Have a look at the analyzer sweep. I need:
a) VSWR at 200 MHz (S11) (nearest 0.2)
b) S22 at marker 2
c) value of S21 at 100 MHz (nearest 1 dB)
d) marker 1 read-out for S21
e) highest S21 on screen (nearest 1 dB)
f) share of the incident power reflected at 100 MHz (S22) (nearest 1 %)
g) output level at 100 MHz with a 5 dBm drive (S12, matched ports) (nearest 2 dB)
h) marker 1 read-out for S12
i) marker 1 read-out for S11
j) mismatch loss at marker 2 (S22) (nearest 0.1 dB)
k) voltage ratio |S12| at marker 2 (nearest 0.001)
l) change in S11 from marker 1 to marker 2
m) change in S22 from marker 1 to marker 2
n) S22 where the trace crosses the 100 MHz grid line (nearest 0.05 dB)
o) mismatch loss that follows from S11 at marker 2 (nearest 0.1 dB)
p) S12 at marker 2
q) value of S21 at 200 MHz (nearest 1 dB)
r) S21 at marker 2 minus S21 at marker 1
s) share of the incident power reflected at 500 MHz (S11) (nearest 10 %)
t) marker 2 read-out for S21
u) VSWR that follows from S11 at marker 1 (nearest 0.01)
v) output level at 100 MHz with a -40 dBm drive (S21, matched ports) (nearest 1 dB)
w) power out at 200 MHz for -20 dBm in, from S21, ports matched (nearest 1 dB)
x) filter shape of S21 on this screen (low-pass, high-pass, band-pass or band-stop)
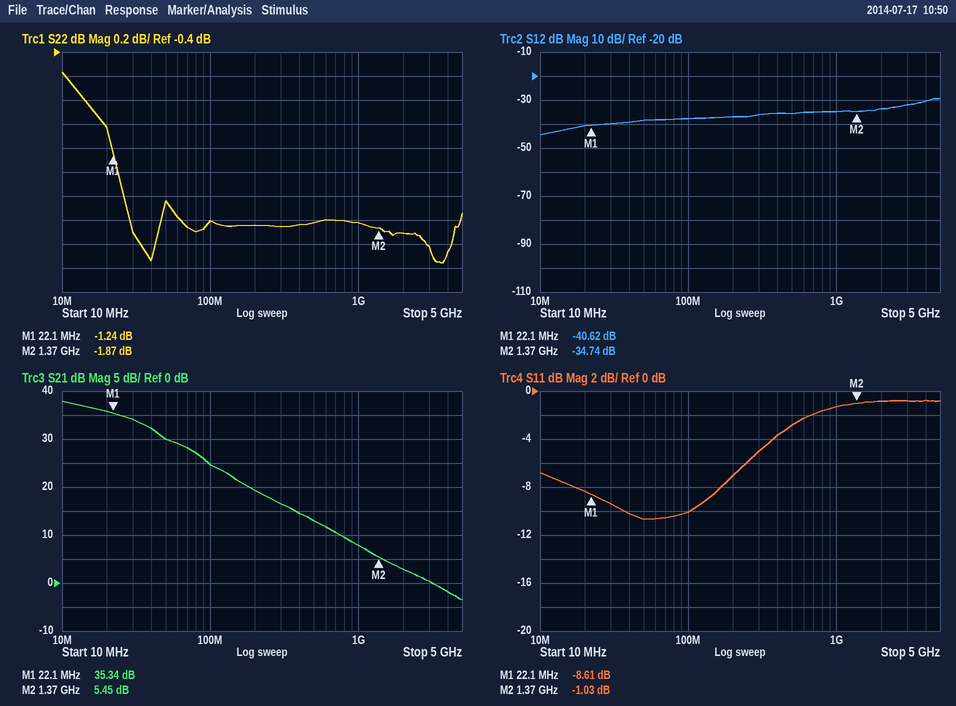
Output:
2.6
-1.87 dB
25 dB
35.34 dB
38 dB
66 %
-32 dBm
-40.62 dB
-8.61 dB
4.6 dB
0.018
7.58 dB
-0.63 dB
-1.80 dB
6.8 dB
-34.74 dB
19 dB
-29.89 dB
50 %
5.45 dB
2.18
-15 dBm
-1 dBm
low-pass
